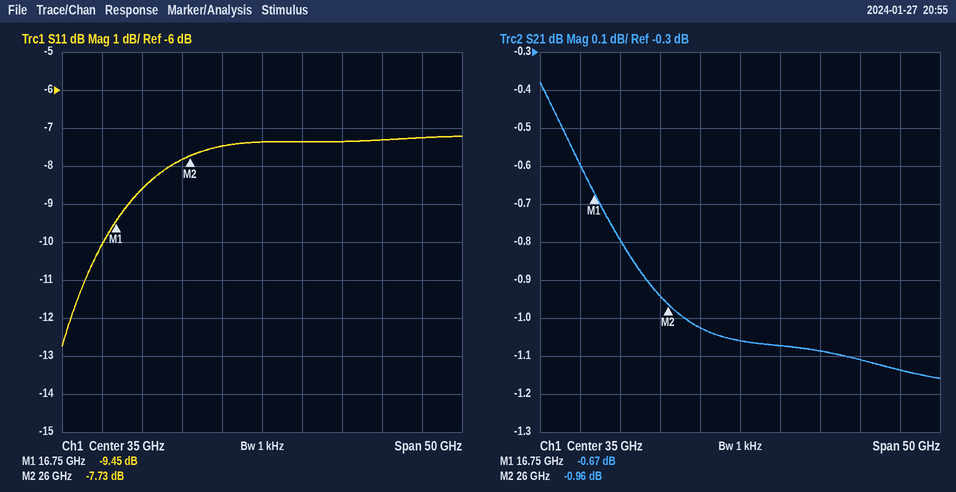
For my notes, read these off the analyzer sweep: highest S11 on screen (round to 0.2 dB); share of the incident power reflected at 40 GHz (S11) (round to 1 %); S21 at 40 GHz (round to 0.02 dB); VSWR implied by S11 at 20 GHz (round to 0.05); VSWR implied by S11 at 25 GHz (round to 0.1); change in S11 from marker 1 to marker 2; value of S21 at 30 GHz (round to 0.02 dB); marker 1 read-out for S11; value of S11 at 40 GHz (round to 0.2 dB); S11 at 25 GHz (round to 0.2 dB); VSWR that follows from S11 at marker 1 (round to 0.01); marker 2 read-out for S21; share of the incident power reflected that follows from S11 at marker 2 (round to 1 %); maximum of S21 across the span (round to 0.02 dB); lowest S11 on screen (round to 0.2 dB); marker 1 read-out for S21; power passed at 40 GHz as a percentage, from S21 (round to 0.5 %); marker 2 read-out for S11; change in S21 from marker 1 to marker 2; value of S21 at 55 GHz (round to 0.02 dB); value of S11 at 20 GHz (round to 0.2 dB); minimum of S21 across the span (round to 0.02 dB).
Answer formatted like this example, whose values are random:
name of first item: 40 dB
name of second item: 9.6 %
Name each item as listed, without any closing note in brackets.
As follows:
highest S11 on screen: -7.2 dB
share of the incident power reflected at 40 GHz (S11): 18 %
S21 at 40 GHz: -1.08 dB
VSWR implied by S11 at 20 GHz: 2.20
VSWR implied by S11 at 25 GHz: 2.4
change in S11 from marker 1 to marker 2: 1.72 dB
value of S21 at 30 GHz: -1.02 dB
marker 1 read-out for S11: -9.45 dB
value of S11 at 40 GHz: -7.4 dB
S11 at 25 GHz: -7.8 dB
VSWR that follows from S11 at marker 1: 2.02
marker 2 read-out for S21: -0.96 dB
share of the incident power reflected that follows from S11 at marker 2: 17 %
maximum of S21 across the span: -0.38 dB
lowest S11 on screen: -12.8 dB
marker 1 read-out for S21: -0.67 dB
power passed at 40 GHz as a percentage, from S21: 78.0 %
marker 2 read-out for S11: -7.73 dB
change in S21 from marker 1 to marker 2: -0.29 dB
value of S21 at 55 GHz: -1.14 dB
value of S11 at 20 GHz: -8.6 dB
minimum of S21 across the span: -1.16 dB
